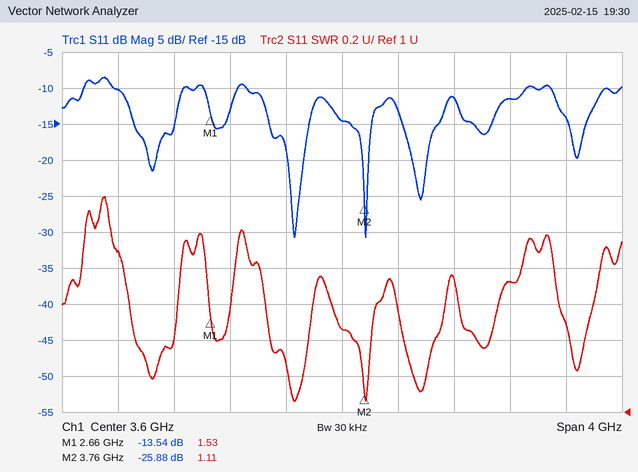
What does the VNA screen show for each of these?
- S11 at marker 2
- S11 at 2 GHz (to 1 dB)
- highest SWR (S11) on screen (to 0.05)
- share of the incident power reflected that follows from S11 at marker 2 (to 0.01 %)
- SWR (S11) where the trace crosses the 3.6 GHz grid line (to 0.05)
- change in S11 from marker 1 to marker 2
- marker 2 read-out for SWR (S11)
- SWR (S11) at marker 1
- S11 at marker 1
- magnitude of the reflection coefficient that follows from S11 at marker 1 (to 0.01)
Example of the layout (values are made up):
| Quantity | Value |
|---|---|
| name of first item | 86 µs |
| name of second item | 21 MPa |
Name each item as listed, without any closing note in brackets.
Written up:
| Quantity | Value |
|---|---|
| S11 at marker 2 | -25.88 dB |
| S11 at 2 GHz | -10 dB |
| highest SWR (S11) on screen | 2.20 |
| share of the incident power reflected that follows from S11 at marker 2 | 0.26 % |
| SWR (S11) where the trace crosses the 3.6 GHz grid line | 1.45 |
| change in S11 from marker 1 to marker 2 | -12.34 dB |
| marker 2 read-out for SWR | 1.11 |
| SWR (S11) at marker 1 | 1.53 |
| S11 at marker 1 | -13.54 dB |
| magnitude of the reflection coefficient that follows from S11 at marker 1 | 0.21 |
